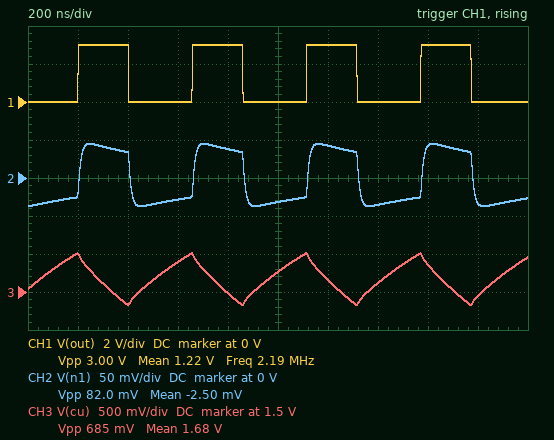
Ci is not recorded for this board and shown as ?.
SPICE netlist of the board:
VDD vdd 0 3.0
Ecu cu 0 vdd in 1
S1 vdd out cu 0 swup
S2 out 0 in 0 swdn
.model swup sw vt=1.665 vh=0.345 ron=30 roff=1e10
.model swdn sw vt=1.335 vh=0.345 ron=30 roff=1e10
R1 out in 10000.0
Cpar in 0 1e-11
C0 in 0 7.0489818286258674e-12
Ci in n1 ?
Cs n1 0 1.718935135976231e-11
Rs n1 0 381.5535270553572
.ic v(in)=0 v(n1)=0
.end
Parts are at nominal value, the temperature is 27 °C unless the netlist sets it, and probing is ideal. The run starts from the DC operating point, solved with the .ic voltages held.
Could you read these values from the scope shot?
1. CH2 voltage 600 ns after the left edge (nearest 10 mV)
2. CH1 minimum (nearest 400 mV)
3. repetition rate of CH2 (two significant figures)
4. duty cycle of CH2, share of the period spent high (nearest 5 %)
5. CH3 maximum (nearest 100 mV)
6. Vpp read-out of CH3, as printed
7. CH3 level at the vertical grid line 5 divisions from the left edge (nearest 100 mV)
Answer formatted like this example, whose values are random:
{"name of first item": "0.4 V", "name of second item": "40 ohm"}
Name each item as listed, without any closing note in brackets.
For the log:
{"CH2 voltage 600 ns after the left edge": "-30 mV", "CH1 minimum": "0 V", "repetition rate of CH2": "2.2 MHz", "duty cycle of CH2, share of the period spent high": "45 %", "CH3 maximum": "2.0 V", "Vpp read-out of CH3, as printed": "685 mV", "CH3 level at the vertical grid line 5 divisions from the left edge": "1.8 V"}
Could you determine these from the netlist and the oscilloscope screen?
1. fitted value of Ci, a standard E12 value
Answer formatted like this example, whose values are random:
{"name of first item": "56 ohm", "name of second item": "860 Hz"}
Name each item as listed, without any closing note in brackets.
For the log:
{"fitted value of Ci, a standard E12 value": "33 pF"}
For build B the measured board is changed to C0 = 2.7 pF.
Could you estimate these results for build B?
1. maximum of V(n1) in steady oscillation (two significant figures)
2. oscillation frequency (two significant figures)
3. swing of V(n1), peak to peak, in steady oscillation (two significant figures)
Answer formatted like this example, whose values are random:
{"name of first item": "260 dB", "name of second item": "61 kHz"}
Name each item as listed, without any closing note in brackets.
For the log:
{"maximum of V(n1) in steady oscillation": "49 mV", "oscillation frequency": "2.4 MHz", "swing of V(n1), peak to peak, in steady oscillation": "89 mV"}
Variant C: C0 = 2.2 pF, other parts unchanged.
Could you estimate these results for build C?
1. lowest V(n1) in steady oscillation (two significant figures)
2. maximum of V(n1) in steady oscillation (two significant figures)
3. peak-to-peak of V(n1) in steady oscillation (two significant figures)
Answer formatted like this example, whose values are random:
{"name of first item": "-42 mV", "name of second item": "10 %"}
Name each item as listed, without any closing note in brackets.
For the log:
{"lowest V(n1) in steady oscillation": "-41 mV", "maximum of V(n1) in steady oscillation": "49 mV", "peak-to-peak of V(n1) in steady oscillation": "90 mV"}
